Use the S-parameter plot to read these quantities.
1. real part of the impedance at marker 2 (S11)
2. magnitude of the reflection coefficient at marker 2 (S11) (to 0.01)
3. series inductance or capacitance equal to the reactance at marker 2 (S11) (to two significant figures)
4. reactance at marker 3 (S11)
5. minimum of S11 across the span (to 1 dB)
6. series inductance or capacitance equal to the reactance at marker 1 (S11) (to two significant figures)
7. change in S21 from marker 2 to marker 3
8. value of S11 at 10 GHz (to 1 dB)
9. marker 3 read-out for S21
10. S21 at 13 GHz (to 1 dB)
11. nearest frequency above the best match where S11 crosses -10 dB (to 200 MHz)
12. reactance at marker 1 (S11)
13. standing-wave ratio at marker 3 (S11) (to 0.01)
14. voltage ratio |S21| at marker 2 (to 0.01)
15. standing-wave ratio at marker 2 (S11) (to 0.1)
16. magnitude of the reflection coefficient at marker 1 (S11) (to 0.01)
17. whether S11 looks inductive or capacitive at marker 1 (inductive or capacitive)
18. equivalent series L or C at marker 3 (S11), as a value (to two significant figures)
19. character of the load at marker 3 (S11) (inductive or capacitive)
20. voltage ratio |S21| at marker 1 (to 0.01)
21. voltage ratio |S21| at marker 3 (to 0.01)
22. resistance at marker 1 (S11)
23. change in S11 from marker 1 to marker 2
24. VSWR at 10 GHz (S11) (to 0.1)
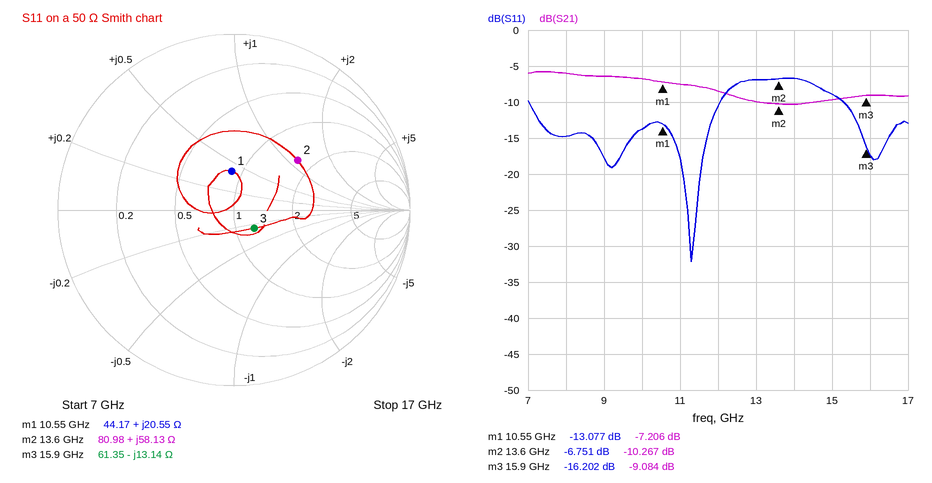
80.98 Ω
0.46
680 pH
-13.14 Ω
-32 dB
310 pH
1.183 dB
-14 dB
-9.084 dB
-10 dB
12.0 GHz
+20.55 Ω
1.37
0.31
2.7
0.22
inductive
760 fF
capacitive
0.44
0.35
44.17 Ω
6.326 dB
1.5
